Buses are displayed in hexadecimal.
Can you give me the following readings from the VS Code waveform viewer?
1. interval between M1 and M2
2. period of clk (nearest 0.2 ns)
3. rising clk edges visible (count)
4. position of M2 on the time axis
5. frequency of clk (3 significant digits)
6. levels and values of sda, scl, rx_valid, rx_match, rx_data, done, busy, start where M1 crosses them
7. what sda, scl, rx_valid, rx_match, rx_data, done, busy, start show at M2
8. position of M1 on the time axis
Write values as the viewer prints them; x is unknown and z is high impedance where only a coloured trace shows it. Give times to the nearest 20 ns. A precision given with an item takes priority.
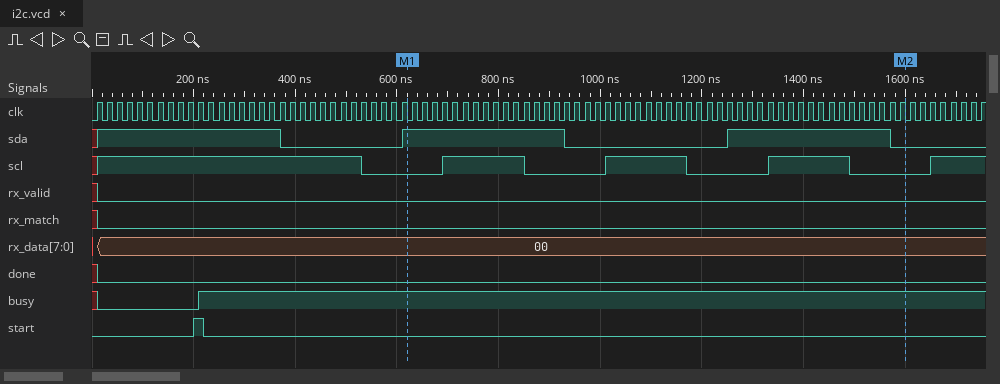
980 ns
20 ns
88
1600 ns
50.0 MHz
sda=1, scl=0, rx_valid=0, rx_match=0, rx_data=00, done=0, busy=1, start=0
sda=0, scl=0, rx_valid=0, rx_match=0, rx_data=00, done=0, busy=1, start=0
620 ns
